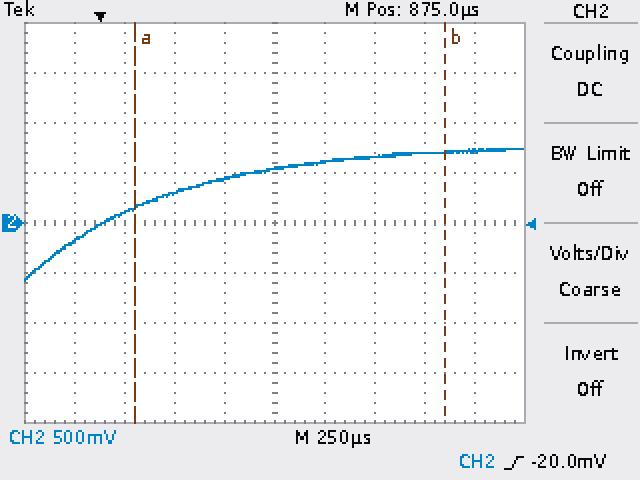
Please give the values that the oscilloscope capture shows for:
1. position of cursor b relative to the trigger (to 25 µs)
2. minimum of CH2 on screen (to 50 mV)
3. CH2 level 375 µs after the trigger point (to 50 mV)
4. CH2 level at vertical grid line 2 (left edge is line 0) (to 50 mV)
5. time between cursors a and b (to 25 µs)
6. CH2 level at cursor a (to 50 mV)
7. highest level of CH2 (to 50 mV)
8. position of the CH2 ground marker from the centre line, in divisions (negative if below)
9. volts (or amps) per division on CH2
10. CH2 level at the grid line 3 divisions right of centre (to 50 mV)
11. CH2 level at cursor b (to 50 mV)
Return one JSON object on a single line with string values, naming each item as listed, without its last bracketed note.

{"position of cursor b relative to the trigger": "+1.725 ms", "minimum of CH2 on screen": "-600 mV", "CH2 level 375 µs after the trigger point": "300 mV", "CH2 level at vertical grid line 2 (left edge is line 0)": "100 mV", "time between cursors a and b": "1.550 ms", "CH2 level at cursor a": "150 mV", "highest level of CH2": "750 mV", "position of the CH2 ground marker from the centre line, in divisions": "0.0 div", "volts (or amps) per division on CH2": "500 mV", "CH2 level at the grid line 3 divisions right of centre": "700 mV", "CH2 level at cursor b": "700 mV"}
